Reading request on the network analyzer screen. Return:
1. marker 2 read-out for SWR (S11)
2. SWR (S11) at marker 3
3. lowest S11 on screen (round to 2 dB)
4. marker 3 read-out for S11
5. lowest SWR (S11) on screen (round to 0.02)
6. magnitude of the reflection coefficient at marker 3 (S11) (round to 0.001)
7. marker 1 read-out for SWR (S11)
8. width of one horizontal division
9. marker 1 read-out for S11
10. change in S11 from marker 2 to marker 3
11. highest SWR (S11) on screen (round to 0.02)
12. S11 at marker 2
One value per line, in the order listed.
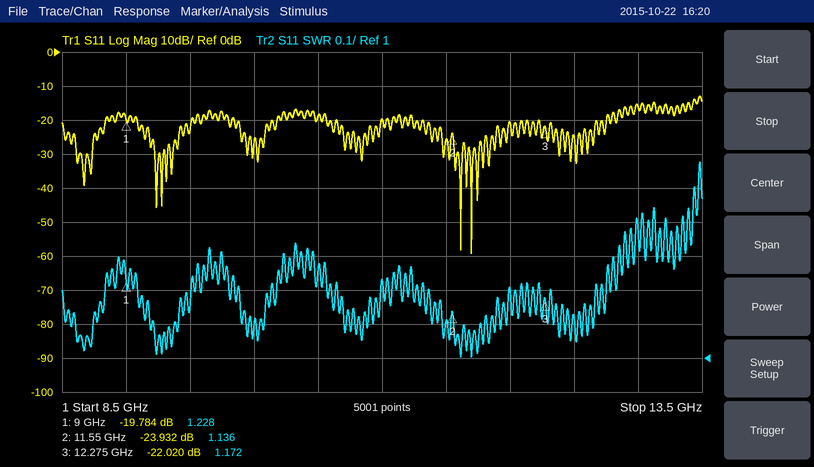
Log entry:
1.136
1.172
-60 dB
-22.020 dB
1.00
0.079
1.228
500 MHz
-19.784 dB
1.912 dB
1.58
-23.932 dB
